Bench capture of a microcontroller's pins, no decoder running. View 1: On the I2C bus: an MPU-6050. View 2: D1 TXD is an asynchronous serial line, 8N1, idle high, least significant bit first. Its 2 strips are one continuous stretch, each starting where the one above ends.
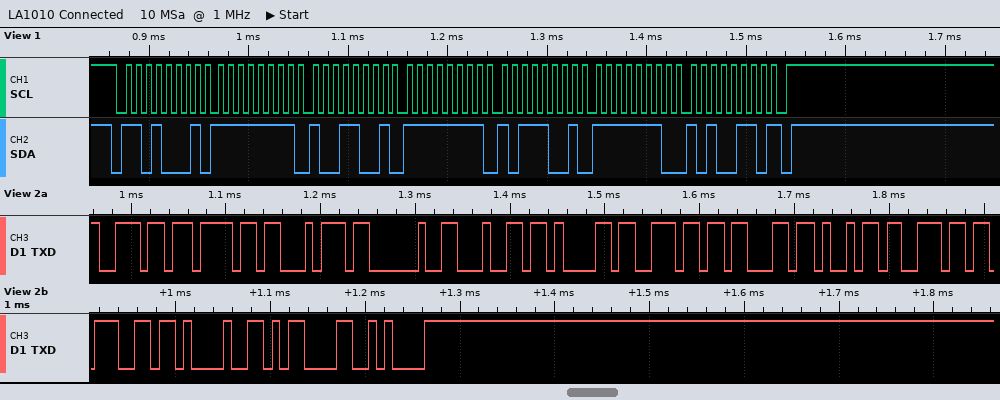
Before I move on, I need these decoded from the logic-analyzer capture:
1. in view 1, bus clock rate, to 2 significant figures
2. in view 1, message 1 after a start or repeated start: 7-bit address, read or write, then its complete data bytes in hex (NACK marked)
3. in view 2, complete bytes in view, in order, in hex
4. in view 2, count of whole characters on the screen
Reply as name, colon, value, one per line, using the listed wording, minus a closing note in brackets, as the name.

in view 1, bus clock rate, to 2 significant figures: 100 kHz
in view 1, message 1 after a start or repeated start: 7-bit address, read or write, then its complete data bytes in hex: 0x68 read: FF 99 FF B9 FE A6 NACK
in view 2, complete bytes in view, in order, in hex: 6E 6F 74 20 64 61 6E 63 69 6E 67 21 0D 0A
in view 2, count of whole characters on the screen: 14
